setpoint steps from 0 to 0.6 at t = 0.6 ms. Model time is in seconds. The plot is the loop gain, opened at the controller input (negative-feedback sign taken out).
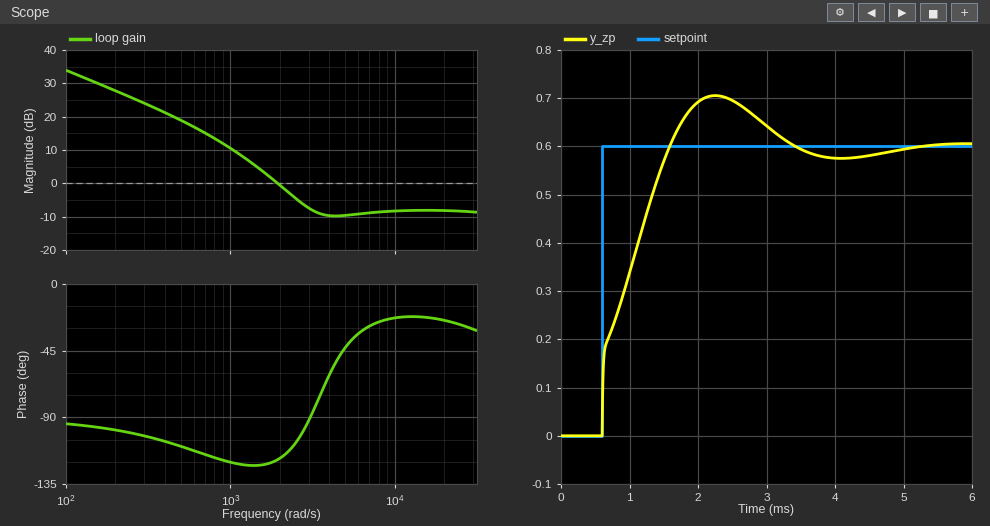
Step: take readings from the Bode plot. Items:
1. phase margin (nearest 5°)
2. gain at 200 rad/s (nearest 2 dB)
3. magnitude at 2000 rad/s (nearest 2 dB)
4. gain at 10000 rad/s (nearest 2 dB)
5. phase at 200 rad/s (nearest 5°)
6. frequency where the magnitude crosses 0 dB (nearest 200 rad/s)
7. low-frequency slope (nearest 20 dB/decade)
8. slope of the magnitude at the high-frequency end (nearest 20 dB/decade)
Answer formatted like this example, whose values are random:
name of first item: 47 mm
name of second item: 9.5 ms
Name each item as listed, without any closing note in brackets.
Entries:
phase margin: 60°
gain at 200 rad/s: 28 dB
magnitude at 2000 rad/s: 0 dB
gain at 10000 rad/s: -8 dB
phase at 200 rad/s: -100°
frequency where the magnitude crosses 0 dB: 2000 rad/s
low-frequency slope: -20 dB/decade
slope of the magnitude at the high-frequency end: 0 dB/decade
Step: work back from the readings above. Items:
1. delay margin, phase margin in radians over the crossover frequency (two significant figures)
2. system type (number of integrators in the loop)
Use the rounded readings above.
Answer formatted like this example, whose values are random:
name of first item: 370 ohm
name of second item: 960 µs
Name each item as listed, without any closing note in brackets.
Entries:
delay margin, phase margin in radians over the crossover frequency: 0.00052 s
system type: 1
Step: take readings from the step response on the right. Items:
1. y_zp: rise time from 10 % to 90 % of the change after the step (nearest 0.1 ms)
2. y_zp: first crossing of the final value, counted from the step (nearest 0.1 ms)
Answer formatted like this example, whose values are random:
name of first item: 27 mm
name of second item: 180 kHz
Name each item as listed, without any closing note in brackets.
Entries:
y_zp: rise time from 10 % to 90 % of the change after the step: 0.8 ms
y_zp: first crossing of the final value, counted from the step: 1.0 ms
